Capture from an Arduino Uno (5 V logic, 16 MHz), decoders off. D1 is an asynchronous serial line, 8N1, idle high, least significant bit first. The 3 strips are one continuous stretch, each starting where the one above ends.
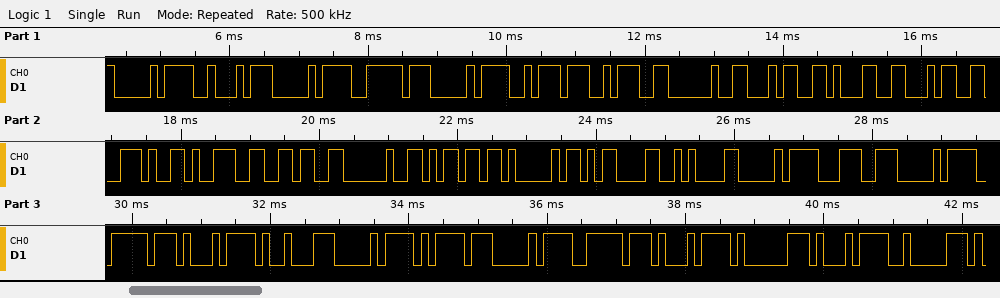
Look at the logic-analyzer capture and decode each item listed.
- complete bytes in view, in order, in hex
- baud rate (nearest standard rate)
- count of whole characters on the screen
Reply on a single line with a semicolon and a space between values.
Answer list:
D0 A2 D0 BE D0 BA 3A 20 34 31 34 2E 39 36 20 6D 41 0D 0A D0 9C D0 BE D1 89 D0 BD D0 BE D1 81 D1 82; 9600 baud; 33
